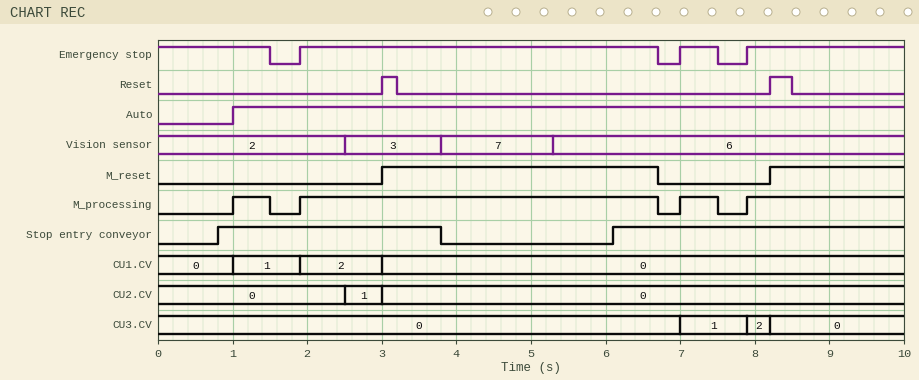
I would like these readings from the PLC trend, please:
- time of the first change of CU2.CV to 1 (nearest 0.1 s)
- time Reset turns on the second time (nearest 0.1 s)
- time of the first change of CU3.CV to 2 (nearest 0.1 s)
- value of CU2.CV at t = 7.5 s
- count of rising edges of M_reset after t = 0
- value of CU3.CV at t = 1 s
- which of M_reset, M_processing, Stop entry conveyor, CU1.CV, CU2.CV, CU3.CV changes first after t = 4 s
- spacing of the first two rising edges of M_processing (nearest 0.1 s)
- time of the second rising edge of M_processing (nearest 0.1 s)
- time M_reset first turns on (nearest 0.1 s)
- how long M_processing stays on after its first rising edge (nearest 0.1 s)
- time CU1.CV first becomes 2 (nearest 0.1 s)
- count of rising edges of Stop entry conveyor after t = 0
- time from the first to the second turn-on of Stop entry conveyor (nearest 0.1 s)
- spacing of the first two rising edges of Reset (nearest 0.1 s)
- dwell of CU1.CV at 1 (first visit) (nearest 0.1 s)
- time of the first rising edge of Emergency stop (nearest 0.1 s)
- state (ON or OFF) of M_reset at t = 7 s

2.5 s
8.2 s
7.9 s
0
2
0
Stop entry conveyor
0.9 s
1.9 s
3.0 s
0.5 s
1.9 s
2
5.3 s
5.2 s
0.9 s
1.9 s
OFF
